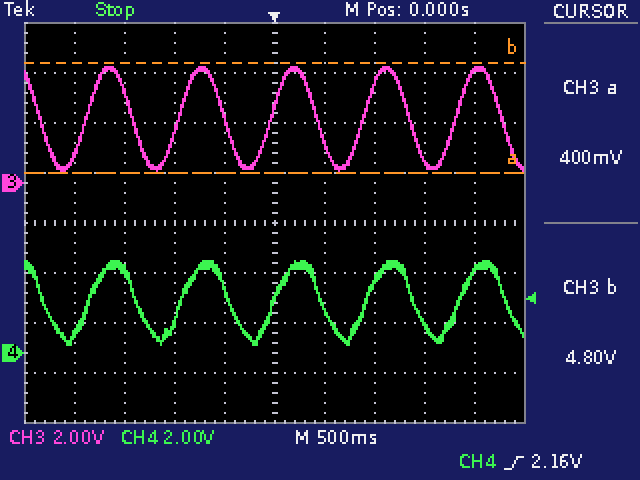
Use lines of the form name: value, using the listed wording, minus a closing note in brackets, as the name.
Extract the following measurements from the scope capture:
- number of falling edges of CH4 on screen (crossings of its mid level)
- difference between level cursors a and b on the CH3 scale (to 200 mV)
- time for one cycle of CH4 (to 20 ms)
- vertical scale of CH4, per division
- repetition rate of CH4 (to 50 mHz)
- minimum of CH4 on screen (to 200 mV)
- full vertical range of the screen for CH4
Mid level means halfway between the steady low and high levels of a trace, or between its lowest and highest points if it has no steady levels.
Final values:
number of falling edges of CH4 on screen: 6
difference between level cursors a and b on the CH3 scale: 4.4 V
time for one cycle of CH4: 920 ms
vertical scale of CH4, per division: 2 V
repetition rate of CH4: 1.10 Hz
minimum of CH4 on screen: 400 mV
full vertical range of the screen for CH4: 16 V
